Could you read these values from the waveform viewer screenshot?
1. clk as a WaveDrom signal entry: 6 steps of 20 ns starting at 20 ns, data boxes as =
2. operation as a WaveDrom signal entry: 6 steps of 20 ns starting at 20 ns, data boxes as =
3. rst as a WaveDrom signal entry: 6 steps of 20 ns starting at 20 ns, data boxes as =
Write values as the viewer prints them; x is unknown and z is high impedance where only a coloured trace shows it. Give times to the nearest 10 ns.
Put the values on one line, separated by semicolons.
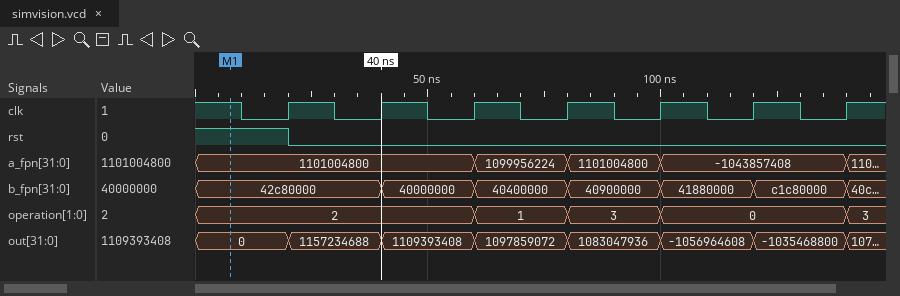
{name: 'clk', wave: 'p.....'}; {name: 'operation', wave: '=.===.', data: '2 1 3 0'}; {name: 'rst', wave: '0.....'}
